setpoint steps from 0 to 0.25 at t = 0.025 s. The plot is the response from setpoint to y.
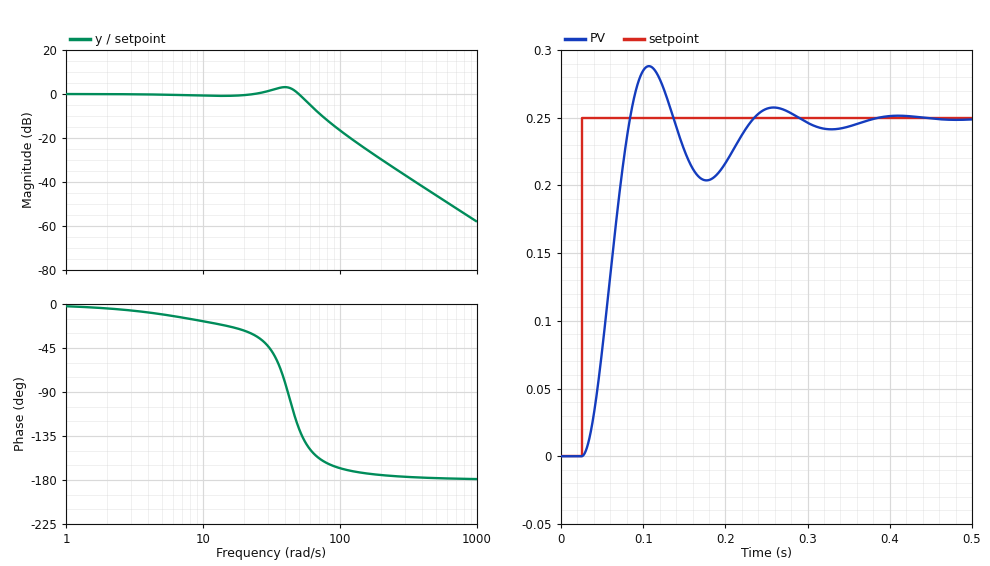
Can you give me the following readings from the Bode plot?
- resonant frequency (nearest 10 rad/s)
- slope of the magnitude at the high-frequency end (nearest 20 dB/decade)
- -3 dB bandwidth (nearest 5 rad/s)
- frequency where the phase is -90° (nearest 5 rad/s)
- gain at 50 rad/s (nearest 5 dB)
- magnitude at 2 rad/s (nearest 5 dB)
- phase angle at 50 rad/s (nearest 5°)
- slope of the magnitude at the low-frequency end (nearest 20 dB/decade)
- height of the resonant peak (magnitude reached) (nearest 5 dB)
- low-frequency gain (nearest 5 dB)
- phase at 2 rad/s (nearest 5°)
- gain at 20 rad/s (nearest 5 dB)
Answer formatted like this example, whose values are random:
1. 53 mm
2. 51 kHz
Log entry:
1. 40 rad/s
2. -40 dB/decade
3. 55 rad/s
4. 40 rad/s
5. 0 dB
6. 0 dB
7. -125°
8. 0 dB/decade
9. 5 dB
10. 0 dB
11. -5°
12. 0 dB
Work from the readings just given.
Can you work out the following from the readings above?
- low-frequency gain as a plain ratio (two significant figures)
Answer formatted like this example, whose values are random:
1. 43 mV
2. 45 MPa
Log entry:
1. 1.0
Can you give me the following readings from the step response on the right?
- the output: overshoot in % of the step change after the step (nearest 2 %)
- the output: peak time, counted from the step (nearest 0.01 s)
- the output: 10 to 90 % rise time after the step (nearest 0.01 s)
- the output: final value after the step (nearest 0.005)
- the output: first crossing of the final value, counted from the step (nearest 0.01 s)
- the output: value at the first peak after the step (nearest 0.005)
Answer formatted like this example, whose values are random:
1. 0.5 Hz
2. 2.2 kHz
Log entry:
1. 16 %
2. 0.08 s
3. 0.04 s
4. 0.250
5. 0.06 s
6. 0.290
